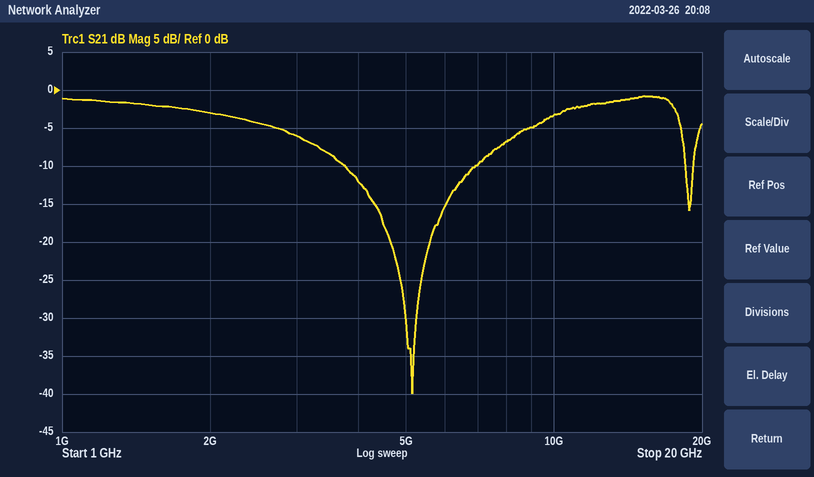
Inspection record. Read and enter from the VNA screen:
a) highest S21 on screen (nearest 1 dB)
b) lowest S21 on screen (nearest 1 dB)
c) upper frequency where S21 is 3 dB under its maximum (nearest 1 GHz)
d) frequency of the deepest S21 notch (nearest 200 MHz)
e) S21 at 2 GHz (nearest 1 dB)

-1 dB
-40 dB
18 GHz
5.2 GHz
-3 dB
